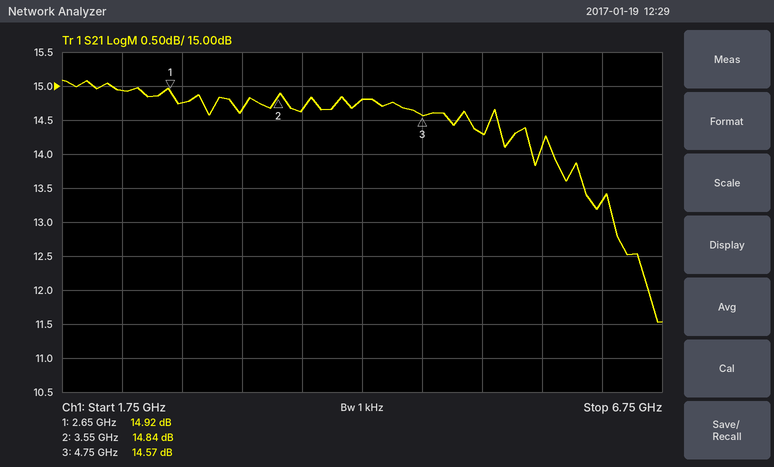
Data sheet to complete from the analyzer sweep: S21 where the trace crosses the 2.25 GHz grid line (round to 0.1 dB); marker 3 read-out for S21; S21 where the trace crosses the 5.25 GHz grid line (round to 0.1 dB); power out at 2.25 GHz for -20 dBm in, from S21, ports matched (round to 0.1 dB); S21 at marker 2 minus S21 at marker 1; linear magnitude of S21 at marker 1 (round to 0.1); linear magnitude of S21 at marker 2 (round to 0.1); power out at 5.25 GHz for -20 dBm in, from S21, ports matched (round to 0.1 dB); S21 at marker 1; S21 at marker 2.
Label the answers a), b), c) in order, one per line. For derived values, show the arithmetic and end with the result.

a) 14.9 dB
b) 14.57 dB
c) 14.3 dB
d) -20 dBm + (14.9 dB) = -5.1 dBm
e) 14.84 − (14.92) = -0.08 dB
f) 10^(14.92/20) ≈ 5.6
g) 10^(14.84/20) ≈ 5.5
h) -20 dBm + (14.3 dB) = -5.7 dBm
i) 14.92 dB
j) 14.84 dB
